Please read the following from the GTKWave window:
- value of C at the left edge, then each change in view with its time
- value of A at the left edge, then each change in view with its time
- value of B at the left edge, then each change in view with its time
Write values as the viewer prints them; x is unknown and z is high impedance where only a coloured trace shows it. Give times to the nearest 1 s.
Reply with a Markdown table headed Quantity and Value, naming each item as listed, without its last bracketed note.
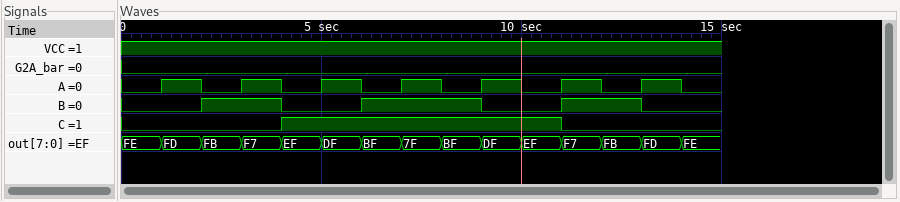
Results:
| Quantity | Value |
|---|---|
| value of C at the left edge, then each change in view with its time | 0, 1 at 4 s, 0 at 11 s |
| value of A at the left edge, then each change in view with its time | 0, 1 at 1 s, 0 at 2 s, 1 at 3 s, 0 at 4 s, 1 at 5 s, 0 at 6 s, 1 at 7 s, 0 at 8 s, 1 at 9 s, 0 at 10 s, 1 at 11 s, 0 at 12 s, 1 at 13 s, 0 at 14 s |
| value of B at the left edge, then each change in view with its time | 0, 1 at 2 s, 0 at 4 s, 1 at 6 s, 0 at 9 s, 1 at 11 s, 0 at 13 s |
